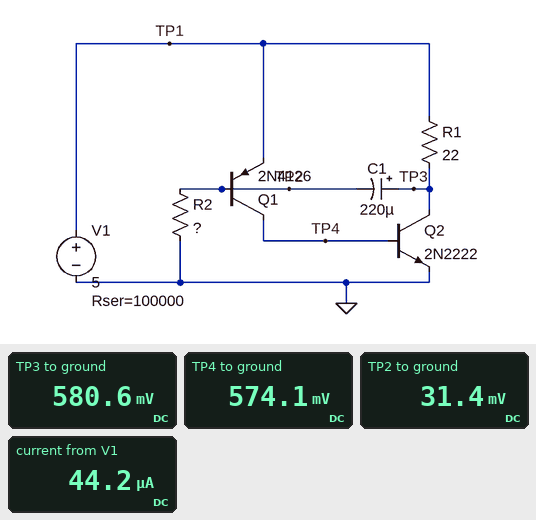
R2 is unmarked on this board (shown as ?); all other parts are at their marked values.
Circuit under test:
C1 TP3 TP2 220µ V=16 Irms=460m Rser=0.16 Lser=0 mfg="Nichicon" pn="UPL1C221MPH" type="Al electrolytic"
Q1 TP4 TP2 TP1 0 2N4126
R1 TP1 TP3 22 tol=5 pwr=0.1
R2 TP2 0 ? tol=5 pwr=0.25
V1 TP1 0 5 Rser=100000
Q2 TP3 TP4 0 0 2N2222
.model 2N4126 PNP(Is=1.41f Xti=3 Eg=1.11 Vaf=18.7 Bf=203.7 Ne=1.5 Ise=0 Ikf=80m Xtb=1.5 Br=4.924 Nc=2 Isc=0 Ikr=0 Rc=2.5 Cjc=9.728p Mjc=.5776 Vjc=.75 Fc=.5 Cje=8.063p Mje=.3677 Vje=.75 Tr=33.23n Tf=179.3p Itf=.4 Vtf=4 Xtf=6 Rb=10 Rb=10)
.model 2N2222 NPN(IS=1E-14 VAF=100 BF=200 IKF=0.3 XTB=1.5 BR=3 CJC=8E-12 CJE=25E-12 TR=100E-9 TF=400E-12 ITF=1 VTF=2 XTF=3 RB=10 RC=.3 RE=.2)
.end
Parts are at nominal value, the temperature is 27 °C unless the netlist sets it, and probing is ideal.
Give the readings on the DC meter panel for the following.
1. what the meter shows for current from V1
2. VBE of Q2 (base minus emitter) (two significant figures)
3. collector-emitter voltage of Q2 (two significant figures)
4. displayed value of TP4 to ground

44.2 µA
570 mV
580 mV
574.1 mV
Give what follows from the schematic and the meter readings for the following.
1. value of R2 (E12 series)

82 kΩ
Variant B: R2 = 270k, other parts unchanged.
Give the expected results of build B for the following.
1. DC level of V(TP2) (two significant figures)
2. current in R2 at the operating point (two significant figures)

50 mV
190 nA
